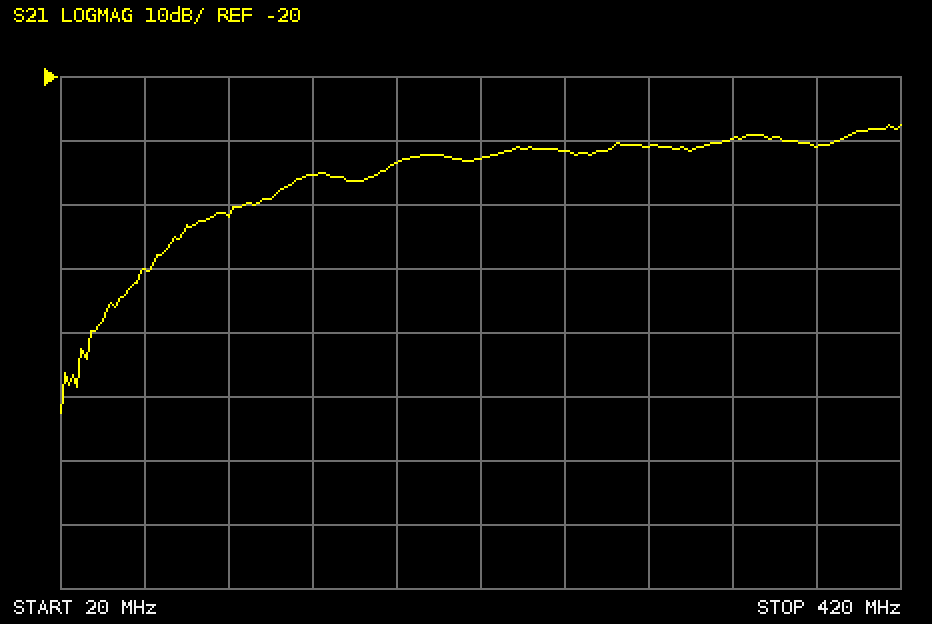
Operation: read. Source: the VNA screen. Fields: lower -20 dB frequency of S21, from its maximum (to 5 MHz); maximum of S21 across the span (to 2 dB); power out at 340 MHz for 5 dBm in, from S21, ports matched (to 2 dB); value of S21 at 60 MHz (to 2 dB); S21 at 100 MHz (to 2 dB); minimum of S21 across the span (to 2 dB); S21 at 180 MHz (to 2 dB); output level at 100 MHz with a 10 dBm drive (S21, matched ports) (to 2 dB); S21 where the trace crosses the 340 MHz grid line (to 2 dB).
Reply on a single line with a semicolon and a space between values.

70 MHz; -28 dB; -24 dBm; -50 dB; -42 dB; -72 dB; -34 dB; -32 dBm; -30 dB
